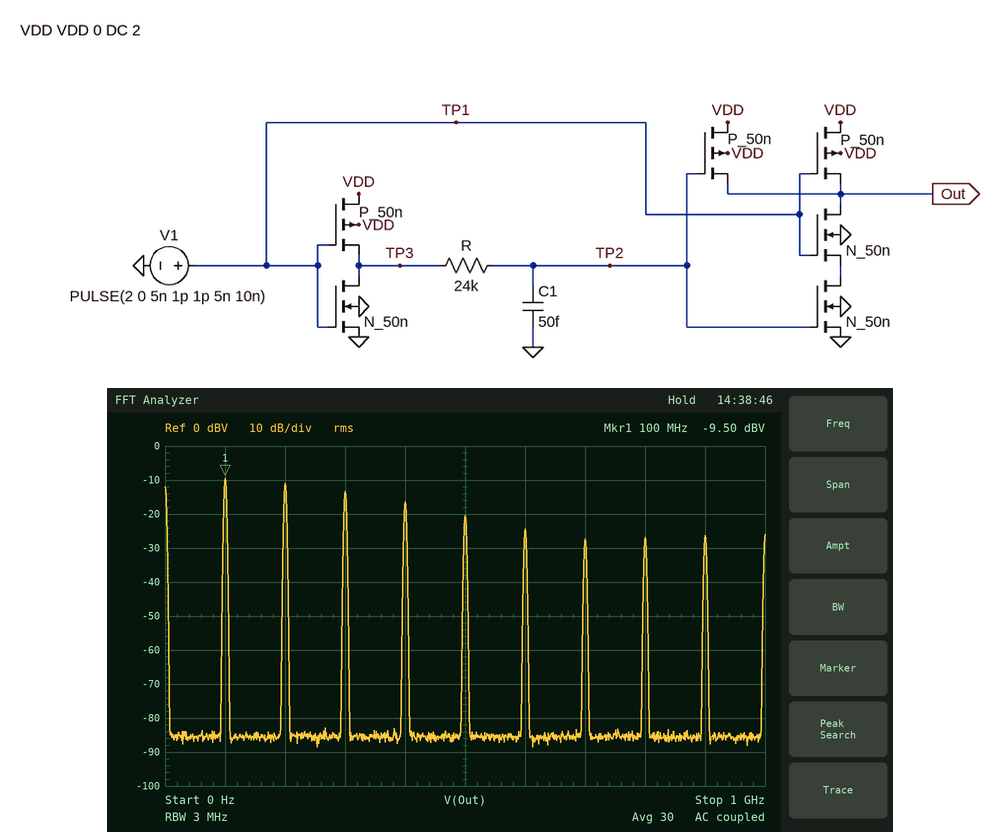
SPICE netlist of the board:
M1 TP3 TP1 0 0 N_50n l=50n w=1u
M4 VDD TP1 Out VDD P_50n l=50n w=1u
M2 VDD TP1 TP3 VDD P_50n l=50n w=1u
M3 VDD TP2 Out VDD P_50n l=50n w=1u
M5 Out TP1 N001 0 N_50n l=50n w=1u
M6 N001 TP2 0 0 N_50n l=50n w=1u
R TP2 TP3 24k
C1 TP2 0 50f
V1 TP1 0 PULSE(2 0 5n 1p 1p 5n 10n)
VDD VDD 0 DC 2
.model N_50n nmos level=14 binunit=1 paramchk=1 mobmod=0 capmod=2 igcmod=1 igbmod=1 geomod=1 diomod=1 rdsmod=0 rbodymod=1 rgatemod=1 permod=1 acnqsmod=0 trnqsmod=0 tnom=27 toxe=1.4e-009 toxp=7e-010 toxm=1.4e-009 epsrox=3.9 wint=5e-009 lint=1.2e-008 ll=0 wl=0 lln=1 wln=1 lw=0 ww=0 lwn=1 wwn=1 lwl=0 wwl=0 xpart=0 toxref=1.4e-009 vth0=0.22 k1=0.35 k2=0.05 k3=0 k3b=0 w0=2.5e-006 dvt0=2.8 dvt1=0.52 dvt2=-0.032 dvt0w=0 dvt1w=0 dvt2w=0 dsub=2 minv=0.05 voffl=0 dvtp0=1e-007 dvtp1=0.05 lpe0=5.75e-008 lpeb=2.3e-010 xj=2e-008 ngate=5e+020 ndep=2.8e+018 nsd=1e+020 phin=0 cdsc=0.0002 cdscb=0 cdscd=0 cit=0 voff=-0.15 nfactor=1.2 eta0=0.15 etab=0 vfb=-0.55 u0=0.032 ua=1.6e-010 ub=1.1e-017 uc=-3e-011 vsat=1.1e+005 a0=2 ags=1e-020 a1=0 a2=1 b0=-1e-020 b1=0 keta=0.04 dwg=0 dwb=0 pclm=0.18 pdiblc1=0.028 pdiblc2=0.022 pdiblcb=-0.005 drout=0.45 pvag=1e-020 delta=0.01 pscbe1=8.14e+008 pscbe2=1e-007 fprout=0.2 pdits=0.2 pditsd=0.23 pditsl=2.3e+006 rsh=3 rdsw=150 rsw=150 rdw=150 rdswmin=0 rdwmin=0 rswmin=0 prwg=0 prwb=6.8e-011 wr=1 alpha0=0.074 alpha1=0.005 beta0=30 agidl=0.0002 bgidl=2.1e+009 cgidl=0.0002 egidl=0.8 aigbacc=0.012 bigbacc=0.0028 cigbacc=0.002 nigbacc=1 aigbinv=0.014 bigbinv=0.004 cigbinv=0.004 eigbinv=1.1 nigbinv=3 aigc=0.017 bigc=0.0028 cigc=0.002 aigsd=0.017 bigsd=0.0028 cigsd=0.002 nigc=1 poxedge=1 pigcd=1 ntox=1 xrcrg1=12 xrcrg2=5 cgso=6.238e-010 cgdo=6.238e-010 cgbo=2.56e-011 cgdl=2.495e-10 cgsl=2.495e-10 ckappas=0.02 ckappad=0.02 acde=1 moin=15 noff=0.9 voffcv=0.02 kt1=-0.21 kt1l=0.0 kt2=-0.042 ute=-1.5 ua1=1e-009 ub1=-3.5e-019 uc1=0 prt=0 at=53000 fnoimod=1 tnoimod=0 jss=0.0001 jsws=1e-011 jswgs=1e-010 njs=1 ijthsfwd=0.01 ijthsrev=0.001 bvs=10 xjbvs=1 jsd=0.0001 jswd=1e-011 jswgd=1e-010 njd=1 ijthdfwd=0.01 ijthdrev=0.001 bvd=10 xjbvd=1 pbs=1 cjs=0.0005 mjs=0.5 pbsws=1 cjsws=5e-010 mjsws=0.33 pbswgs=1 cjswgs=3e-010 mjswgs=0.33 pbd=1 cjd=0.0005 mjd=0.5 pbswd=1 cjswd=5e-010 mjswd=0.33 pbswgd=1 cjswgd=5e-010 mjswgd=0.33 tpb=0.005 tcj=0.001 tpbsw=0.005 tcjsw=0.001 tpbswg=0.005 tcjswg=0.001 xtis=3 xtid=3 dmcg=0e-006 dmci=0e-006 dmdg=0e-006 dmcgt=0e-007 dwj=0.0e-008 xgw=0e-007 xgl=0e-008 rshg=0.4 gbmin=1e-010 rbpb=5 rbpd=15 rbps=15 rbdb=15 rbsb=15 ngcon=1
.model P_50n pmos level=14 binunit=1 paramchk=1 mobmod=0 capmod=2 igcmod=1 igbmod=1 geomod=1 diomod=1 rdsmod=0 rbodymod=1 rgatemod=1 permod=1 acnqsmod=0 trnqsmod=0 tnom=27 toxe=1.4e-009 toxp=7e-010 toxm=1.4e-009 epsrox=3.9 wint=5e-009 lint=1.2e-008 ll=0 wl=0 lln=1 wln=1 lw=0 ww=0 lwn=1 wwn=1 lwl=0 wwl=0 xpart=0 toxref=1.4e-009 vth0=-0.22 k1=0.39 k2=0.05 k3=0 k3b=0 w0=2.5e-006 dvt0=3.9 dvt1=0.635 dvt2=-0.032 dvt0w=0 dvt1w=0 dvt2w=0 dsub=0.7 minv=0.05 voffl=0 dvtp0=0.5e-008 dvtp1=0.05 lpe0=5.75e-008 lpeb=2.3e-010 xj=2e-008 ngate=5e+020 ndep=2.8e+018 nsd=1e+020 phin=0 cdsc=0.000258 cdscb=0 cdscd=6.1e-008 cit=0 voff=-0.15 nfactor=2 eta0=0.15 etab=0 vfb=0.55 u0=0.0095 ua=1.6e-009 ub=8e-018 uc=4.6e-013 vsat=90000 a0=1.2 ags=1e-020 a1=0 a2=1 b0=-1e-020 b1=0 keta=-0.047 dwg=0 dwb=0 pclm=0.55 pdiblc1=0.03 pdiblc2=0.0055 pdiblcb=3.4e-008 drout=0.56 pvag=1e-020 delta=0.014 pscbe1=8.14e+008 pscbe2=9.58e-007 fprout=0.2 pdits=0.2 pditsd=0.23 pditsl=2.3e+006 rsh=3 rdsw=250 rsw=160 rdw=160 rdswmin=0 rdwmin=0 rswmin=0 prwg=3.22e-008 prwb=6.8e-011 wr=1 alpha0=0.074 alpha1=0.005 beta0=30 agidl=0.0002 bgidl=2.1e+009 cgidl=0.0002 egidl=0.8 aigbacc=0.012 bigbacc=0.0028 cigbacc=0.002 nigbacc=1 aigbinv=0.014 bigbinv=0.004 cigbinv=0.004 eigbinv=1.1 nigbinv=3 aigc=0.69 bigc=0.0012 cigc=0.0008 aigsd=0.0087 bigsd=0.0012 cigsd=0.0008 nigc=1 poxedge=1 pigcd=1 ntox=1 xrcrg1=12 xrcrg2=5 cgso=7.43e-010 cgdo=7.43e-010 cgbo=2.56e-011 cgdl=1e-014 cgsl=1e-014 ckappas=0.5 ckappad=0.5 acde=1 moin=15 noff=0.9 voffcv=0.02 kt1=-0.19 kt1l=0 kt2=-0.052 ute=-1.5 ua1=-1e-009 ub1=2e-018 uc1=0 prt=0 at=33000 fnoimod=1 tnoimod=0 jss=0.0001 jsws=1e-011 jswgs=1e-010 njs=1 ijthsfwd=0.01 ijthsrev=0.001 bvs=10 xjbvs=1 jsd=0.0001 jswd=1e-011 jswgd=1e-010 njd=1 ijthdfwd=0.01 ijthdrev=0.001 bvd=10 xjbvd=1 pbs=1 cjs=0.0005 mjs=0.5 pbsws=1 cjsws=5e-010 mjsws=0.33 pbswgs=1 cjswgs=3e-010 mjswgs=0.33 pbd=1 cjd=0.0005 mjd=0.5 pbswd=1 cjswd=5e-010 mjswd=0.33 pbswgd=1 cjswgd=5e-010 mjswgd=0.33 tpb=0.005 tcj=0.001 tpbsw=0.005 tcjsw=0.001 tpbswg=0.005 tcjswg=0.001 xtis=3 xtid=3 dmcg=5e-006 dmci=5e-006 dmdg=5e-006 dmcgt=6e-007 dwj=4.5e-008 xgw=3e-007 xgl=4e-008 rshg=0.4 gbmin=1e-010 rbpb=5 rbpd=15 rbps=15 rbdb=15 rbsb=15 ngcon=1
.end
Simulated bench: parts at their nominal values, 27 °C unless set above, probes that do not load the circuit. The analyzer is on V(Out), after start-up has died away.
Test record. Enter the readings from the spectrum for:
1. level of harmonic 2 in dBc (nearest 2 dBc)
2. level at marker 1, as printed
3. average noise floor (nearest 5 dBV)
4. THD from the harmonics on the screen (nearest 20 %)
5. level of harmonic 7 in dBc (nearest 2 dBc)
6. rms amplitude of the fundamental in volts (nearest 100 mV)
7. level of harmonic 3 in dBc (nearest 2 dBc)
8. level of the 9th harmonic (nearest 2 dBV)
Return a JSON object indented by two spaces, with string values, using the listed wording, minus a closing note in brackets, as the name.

{
  "level of harmonic 2 in dBc": "-2 dBc",
  "level at marker 1, as printed": "-9.50 dBV",
  "average noise floor": "-85 dBV",
  "THD from the harmonics on the screen": "120 %",
  "level of harmonic 7 in dBc": "-18 dBc",
  "rms amplitude of the fundamental in volts": "300 mV",
  "level of harmonic 3 in dBc": "-4 dBc",
  "level of the 9th harmonic": "-26 dBV"
}
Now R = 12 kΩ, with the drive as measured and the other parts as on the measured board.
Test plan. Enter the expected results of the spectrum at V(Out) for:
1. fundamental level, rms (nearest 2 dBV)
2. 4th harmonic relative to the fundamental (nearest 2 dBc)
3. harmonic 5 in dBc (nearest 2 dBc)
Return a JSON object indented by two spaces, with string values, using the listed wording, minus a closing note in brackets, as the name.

{
  "fundamental level, rms": "-14 dBV",
  "4th harmonic relative to the fundamental": "-2 dBc",
  "harmonic 5 in dBc": "-4 dBc"
}
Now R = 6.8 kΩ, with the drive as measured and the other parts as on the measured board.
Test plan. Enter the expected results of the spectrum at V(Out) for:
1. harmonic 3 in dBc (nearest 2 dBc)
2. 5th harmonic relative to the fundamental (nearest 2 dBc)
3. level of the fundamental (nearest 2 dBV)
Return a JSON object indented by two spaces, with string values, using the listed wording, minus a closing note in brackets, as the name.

{
  "harmonic 3 in dBc": "0 dBc",
  "5th harmonic relative to the fundamental": "-2 dBc",
  "level of the fundamental": "-18 dBV"
}
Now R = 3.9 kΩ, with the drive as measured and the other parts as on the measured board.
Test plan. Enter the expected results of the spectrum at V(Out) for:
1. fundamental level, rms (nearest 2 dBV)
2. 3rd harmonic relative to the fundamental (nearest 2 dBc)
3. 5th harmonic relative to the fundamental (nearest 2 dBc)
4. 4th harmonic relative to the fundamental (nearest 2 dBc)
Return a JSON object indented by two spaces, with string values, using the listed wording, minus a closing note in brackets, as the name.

{
  "fundamental level, rms": "-22 dBV",
  "3rd harmonic relative to the fundamental": "0 dBc",
  "5th harmonic relative to the fundamental": "0 dBc",
  "4th harmonic relative to the fundamental": "0 dBc"
}
